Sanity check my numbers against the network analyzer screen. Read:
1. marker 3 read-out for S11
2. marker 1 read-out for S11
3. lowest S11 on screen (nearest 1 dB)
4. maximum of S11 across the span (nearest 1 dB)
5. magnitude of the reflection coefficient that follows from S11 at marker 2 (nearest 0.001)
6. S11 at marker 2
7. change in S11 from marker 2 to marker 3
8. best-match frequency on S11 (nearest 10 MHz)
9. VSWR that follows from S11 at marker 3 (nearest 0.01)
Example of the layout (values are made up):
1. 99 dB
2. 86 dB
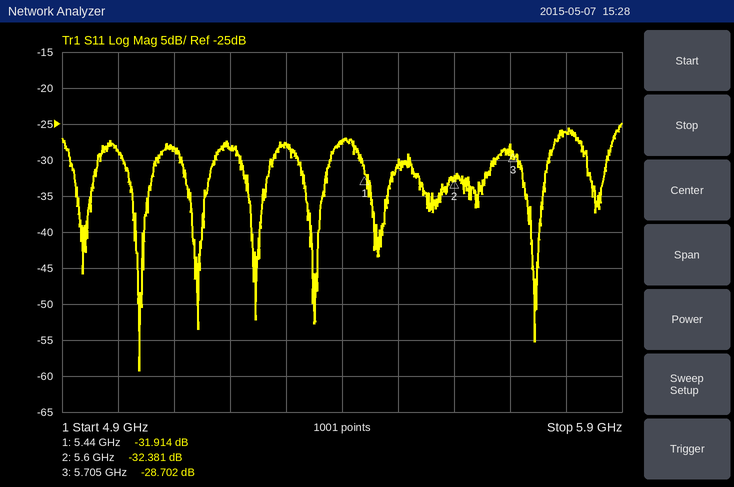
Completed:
1. -28.702 dB
2. -31.914 dB
3. -59 dB
4. -25 dB
5. 0.024
6. -32.381 dB
7. 3.679 dB
8. 5.04 GHz
9. 1.08
